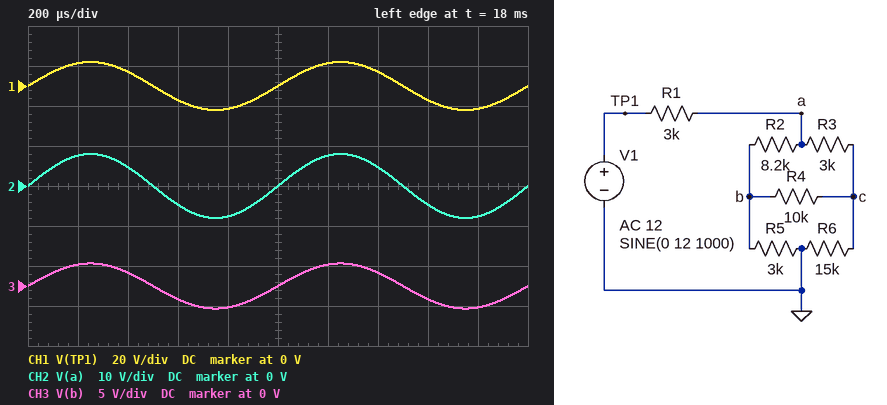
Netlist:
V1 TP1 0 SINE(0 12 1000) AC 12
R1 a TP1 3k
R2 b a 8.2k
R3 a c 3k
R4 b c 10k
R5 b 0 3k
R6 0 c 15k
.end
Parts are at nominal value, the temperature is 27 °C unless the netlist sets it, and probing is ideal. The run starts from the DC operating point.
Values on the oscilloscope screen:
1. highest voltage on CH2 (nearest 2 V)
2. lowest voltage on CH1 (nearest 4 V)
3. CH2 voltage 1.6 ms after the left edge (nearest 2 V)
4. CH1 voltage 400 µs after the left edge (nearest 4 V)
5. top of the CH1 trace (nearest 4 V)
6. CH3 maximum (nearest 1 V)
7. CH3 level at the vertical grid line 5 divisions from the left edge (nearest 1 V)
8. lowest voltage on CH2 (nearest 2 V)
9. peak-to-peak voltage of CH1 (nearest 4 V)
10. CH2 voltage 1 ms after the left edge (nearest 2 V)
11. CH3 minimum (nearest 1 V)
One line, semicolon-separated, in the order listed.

8 V; -12 V; -4 V; 8 V; 12 V; 3 V; 0 V; -8 V; 24 V; 0 V; -3 V
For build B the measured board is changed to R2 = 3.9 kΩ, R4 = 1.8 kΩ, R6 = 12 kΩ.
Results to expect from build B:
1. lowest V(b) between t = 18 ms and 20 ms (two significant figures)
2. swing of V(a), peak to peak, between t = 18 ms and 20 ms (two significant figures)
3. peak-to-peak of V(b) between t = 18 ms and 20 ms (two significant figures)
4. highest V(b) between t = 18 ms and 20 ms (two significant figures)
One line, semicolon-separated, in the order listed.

-3.8 V; 14 V; 7.6 V; 3.8 V
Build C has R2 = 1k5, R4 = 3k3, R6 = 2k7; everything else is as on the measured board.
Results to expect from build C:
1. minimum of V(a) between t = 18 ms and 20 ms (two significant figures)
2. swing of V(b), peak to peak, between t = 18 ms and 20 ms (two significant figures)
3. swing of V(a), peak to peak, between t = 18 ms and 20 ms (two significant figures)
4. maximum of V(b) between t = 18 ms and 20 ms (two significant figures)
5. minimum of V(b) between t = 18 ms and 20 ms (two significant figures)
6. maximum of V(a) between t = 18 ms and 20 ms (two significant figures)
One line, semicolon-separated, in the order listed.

-5.4 V; 6.9 V; 11 V; 3.4 V; -3.4 V; 5.4 V
